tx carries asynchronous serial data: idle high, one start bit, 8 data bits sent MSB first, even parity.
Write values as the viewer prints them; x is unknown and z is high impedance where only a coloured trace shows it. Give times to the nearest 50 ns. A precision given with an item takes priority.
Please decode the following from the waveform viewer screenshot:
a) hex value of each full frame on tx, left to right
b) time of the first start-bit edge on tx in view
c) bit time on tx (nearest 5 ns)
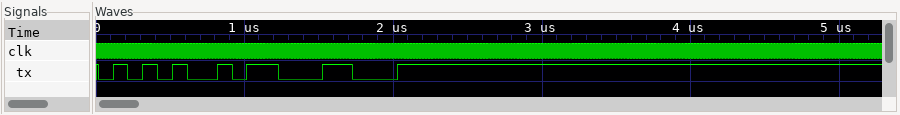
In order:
A9, 31
0 ns
100 ns
